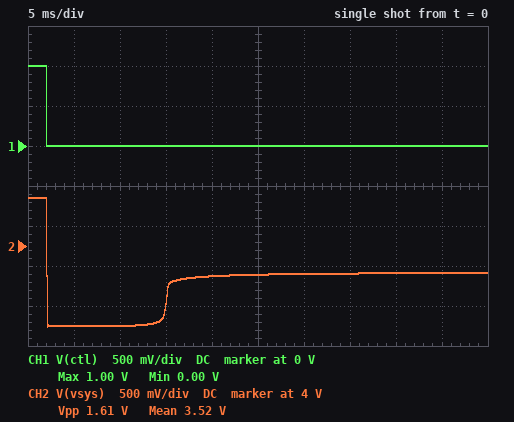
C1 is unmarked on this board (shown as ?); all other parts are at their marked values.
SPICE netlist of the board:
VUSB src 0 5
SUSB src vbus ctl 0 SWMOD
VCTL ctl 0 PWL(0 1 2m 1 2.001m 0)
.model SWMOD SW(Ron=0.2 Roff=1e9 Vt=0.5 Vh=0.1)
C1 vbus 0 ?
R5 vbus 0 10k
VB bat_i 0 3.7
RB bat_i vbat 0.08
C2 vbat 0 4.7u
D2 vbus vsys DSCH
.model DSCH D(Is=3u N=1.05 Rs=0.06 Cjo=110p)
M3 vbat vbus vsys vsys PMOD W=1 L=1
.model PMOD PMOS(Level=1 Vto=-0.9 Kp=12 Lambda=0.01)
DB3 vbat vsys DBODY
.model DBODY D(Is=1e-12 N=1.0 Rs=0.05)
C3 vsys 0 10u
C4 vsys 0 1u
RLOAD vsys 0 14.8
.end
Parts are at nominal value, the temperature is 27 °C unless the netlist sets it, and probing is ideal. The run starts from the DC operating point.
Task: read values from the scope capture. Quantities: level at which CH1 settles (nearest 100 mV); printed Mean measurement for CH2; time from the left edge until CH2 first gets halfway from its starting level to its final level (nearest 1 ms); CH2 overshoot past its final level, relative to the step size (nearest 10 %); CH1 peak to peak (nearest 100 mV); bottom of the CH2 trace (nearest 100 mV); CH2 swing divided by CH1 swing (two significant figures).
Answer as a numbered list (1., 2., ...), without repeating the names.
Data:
1. 0 V
2. 3.52 V
3. 2 ms
4. 70 %
5. 1.0 V
6. 3.0 V
7. 1.6
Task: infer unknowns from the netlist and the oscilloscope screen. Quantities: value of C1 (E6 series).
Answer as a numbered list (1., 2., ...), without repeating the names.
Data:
1. 6.8 µF
